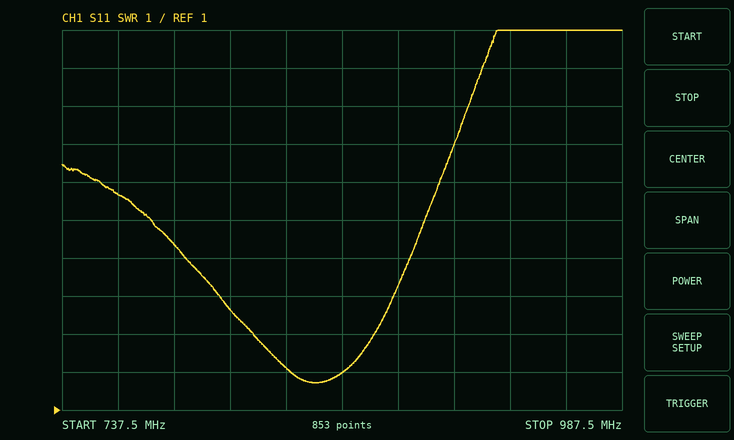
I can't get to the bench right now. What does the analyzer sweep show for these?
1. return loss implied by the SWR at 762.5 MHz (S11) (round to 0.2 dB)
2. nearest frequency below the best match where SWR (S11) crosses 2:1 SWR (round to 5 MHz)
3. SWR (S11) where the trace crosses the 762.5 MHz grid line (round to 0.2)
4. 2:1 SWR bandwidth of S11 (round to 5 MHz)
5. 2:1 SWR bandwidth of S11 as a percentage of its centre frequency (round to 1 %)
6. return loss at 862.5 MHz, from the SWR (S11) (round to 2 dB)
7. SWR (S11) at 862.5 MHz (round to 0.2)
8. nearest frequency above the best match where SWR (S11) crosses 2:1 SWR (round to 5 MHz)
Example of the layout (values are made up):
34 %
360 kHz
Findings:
2.6 dB
840 MHz
6.6
25 MHz
3 %
10 dB
2.0
865 MHz
